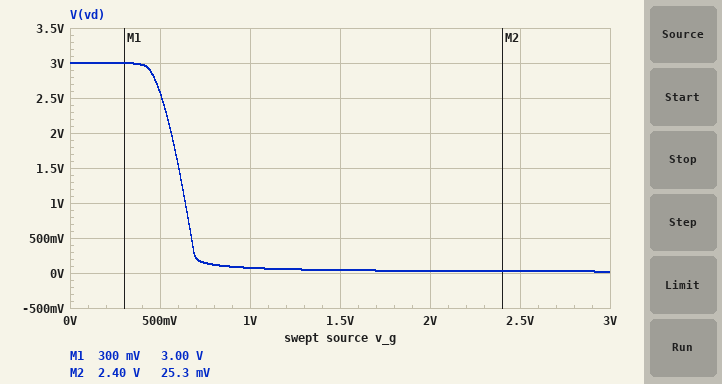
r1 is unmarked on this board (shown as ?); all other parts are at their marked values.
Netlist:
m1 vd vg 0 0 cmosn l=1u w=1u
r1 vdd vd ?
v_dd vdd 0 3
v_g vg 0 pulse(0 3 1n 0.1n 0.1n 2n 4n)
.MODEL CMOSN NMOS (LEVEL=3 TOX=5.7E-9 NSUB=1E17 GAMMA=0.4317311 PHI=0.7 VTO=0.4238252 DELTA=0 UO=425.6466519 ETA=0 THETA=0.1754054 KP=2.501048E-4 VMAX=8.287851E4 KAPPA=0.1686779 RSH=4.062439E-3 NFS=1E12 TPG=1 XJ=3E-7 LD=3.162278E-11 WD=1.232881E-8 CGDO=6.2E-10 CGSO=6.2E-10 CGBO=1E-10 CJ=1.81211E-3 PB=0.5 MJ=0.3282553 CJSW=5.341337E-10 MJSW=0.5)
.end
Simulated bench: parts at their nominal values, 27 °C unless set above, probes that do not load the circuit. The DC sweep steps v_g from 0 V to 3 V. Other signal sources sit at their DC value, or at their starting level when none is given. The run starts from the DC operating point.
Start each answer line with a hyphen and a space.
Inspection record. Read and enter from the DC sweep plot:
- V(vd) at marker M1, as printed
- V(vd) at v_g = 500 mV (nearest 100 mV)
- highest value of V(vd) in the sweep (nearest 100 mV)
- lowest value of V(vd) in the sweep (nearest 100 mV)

- 3.00 V
- 2.6 V
- 3.0 V
- 0 V
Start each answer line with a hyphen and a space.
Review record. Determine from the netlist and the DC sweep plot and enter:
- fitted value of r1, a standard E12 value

- 330 kΩ
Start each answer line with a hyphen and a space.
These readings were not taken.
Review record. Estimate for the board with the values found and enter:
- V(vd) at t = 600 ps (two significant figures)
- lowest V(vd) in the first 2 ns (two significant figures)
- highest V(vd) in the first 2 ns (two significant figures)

- 3.0 V
- 21 mV
- 3.6 V
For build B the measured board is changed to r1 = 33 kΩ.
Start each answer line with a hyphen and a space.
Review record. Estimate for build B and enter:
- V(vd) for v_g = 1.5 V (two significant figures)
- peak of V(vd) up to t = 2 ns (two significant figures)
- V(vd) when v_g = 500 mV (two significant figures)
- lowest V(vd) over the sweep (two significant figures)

- 570 mV
- 3.4 V
- 3.0 V
- 220 mV
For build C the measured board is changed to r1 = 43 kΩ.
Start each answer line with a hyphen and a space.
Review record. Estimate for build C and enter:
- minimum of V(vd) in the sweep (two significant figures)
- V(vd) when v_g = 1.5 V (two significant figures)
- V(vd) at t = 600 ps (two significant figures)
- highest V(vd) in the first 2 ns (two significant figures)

- 170 mV
- 390 mV
- 3.0 V
- 3.4 V
